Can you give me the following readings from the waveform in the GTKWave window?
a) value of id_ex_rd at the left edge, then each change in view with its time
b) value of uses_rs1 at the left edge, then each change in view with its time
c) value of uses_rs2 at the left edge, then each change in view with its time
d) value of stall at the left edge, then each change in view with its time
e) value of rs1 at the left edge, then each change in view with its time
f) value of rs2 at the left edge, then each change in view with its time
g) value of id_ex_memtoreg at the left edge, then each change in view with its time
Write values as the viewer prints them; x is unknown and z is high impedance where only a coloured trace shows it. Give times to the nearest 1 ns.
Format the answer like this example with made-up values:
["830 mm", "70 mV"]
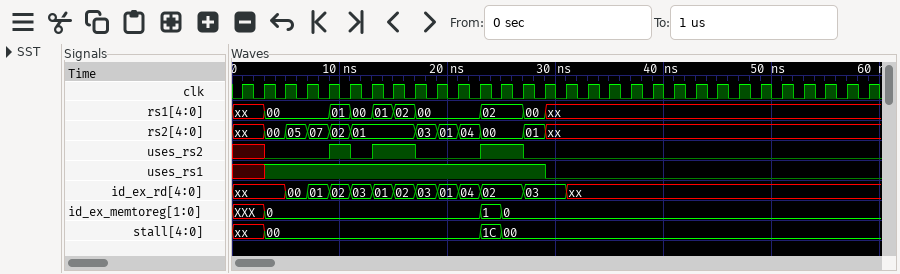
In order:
["xx, 00 at 5 ns, 01 at 7 ns, 02 at 9 ns, 03 at 11 ns, 01 at 13 ns, 02 at 15 ns, 03 at 17 ns, 01 at 19 ns, 04 at 21 ns, 02 at 23 ns, 03 at 27 ns, xx at 31 ns", "x, 1 at 3 ns, 0 at 29 ns", "x, 0 at 3 ns, 1 at 9 ns, 0 at 11 ns, 1 at 13 ns, 0 at 17 ns, 1 at 23 ns, 0 at 27 ns", "xx, 00 at 3 ns, 1C at 23 ns, 00 at 25 ns", "xx, 00 at 3 ns, 01 at 9 ns, 00 at 11 ns, 01 at 13 ns, 02 at 15 ns, 00 at 17 ns, 02 at 23 ns, 00 at 27 ns, xx at 29 ns", "xx, 00 at 3 ns, 05 at 5 ns, 07 at 7 ns, 02 at 9 ns, 01 at 11 ns, 03 at 17 ns, 01 at 19 ns, 04 at 21 ns, 00 at 23 ns, 01 at 27 ns, xx at 29 ns", "XXX, 0 at 3 ns, 1 at 23 ns, 0 at 25 ns"]
